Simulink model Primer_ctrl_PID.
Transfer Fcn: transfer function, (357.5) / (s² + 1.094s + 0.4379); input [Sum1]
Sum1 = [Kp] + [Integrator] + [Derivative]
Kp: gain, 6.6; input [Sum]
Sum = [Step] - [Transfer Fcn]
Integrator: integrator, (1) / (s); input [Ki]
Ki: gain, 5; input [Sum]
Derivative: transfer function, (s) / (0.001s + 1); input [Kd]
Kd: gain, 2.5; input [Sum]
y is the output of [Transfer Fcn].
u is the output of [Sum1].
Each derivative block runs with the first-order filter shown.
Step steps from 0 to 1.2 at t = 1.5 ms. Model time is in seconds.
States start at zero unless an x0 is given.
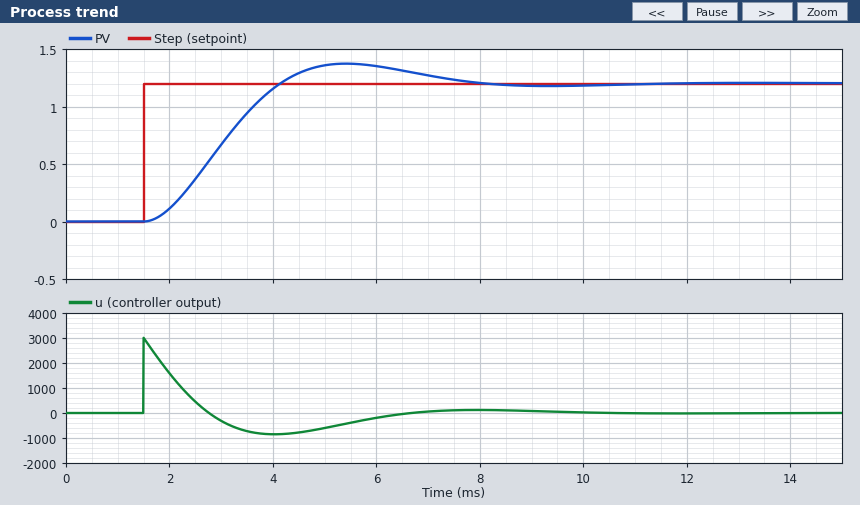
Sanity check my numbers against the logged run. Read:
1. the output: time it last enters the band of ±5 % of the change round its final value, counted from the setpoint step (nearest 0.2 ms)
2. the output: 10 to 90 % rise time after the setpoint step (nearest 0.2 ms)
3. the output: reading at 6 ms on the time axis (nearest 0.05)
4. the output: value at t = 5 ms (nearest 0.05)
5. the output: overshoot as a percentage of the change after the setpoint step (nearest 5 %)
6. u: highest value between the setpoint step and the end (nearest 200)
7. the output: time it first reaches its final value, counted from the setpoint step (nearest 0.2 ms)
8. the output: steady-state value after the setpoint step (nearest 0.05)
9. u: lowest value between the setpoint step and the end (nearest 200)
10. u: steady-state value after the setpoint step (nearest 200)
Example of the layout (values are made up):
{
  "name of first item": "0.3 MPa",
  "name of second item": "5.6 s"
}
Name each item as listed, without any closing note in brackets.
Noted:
{
  "the output: time it last enters the band of ±5 % of the change round its final value, counted from the setpoint step": "5.6 ms",
  "the output: 10 to 90 % rise time after the setpoint step": "1.8 ms",
  "the output: reading at 6 ms on the time axis": "1.35",
  "the output: value at t = 5 ms": "1.35",
  "the output: overshoot as a percentage of the change after the setpoint step": "15 %",
  "u: highest value between the setpoint step and the end": "3000",
  "the output: time it first reaches its final value, counted from the setpoint step": "2.6 ms",
  "the output: steady-state value after the setpoint step": "1.20",
  "u: lowest value between the setpoint step and the end": "-800",
  "u: steady-state value after the setpoint step": "0"
}
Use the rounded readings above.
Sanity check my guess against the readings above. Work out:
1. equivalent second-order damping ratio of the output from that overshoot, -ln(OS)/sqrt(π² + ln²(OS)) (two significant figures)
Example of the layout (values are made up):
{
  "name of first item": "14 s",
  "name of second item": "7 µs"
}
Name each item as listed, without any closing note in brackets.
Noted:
{
  "equivalent second-order damping ratio of the output from that overshoot, -ln(OS)/sqrt(π² + ln²(OS))": "0.52"
}
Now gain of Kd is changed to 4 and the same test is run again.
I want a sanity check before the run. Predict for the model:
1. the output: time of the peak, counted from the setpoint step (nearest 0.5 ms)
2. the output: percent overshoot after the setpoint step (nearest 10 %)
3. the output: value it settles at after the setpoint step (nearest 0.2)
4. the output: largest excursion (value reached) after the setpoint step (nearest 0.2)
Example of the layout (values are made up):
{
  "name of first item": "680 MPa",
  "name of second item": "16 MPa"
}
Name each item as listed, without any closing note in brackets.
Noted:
{
  "the output: time of the peak, counted from the setpoint step": "3.0 ms",
  "the output: percent overshoot after the setpoint step": "20 %",
  "the output: value it settles at after the setpoint step": "1.2",
  "the output: largest excursion (value reached) after the setpoint step": "1.4"
}
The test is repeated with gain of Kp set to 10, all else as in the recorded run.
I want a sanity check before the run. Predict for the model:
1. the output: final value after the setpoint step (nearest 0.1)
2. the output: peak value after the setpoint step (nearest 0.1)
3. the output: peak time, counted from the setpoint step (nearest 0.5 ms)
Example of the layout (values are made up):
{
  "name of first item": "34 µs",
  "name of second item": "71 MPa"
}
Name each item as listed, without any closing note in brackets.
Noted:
{
  "the output: final value after the setpoint step": "1.2",
  "the output: peak value after the setpoint step": "1.4",
  "the output: peak time, counted from the setpoint step": "4.0 ms"
}
